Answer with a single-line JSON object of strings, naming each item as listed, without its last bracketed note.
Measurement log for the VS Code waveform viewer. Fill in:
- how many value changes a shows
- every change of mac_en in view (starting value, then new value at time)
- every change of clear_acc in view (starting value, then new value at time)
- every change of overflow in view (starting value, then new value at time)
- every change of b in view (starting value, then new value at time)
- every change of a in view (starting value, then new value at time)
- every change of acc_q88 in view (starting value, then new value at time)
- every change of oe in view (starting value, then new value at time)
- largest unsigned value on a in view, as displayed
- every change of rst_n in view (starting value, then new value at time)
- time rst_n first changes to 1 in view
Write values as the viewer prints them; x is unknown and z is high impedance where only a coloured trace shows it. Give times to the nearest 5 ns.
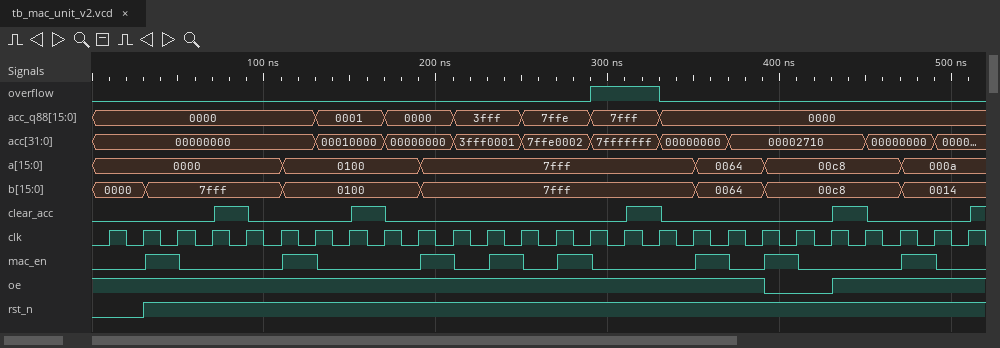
{"how many value changes a shows": "5", "every change of mac_en in view": "0, 1 at 30 ns, 0 at 50 ns, 1 at 110 ns, 0 at 130 ns, 1 at 190 ns, 0 at 210 ns, 1 at 230 ns, 0 at 250 ns, 1 at 270 ns, 0 at 290 ns, 1 at 350 ns, 0 at 370 ns, 1 at 390 ns, 0 at 410 ns, 1 at 470 ns, 0 at 490 ns", "every change of clear_acc in view": "0, 1 at 70 ns, 0 at 90 ns, 1 at 150 ns, 0 at 170 ns, 1 at 310 ns, 0 at 330 ns, 1 at 430 ns, 0 at 450 ns, 1 at 510 ns", "every change of overflow in view": "0, 1 at 290 ns, 0 at 330 ns", "every change of b in view": "0000, 7fff at 30 ns, 0100 at 110 ns, 7fff at 190 ns, 0064 at 350 ns, 00c8 at 390 ns, 0014 at 470 ns", "every change of a in view": "0000, 0100 at 110 ns, 7fff at 190 ns, 0064 at 350 ns, 00c8 at 390 ns, 000a at 470 ns", "every change of acc_q88 in view": "0000, 0001 at 130 ns, 0000 at 170 ns, 3fff at 210 ns, 7ffe at 250 ns, 7fff at 290 ns, 0000 at 330 ns", "every change of oe in view": "1, 0 at 390 ns, 1 at 430 ns", "largest unsigned value on a in view, as displayed": "7fff", "every change of rst_n in view": "0, 1 at 30 ns", "time rst_n first changes to 1 in view": "30 ns"}
